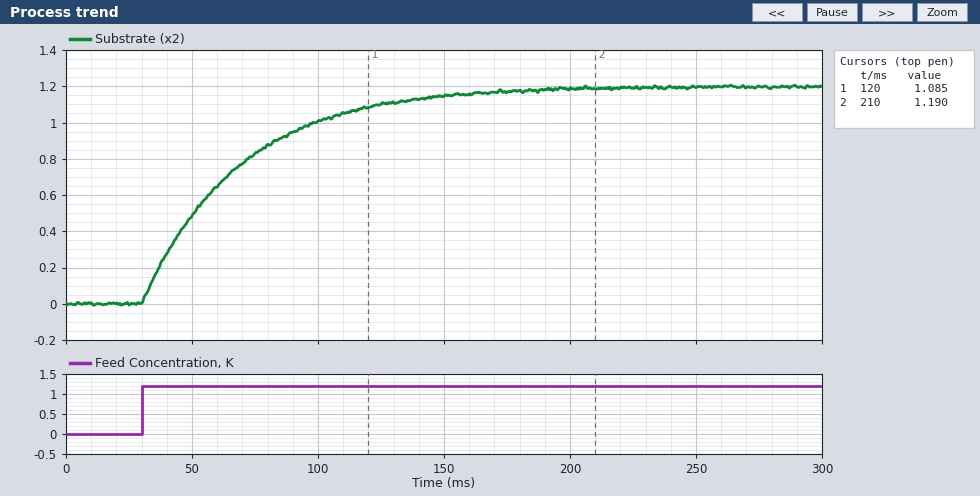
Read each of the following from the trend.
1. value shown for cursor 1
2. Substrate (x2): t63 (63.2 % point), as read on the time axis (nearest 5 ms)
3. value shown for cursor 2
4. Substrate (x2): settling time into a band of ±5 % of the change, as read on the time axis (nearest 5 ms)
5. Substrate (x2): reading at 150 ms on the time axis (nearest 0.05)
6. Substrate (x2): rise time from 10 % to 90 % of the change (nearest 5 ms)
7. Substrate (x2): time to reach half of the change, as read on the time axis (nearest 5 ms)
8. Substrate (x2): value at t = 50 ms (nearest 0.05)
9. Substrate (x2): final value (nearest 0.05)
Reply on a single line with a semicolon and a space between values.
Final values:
1.085; 70 ms; 1.190; 145 ms; 1.15; 85 ms; 55 ms; 0.50; 1.20
